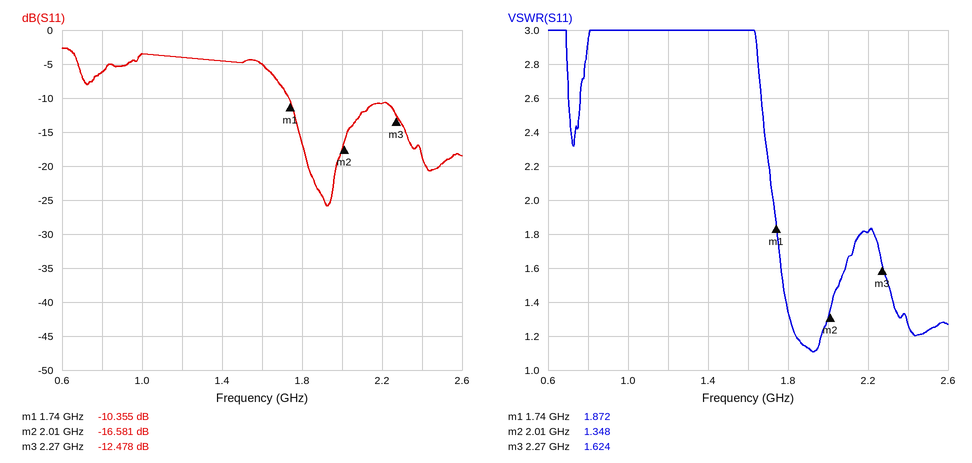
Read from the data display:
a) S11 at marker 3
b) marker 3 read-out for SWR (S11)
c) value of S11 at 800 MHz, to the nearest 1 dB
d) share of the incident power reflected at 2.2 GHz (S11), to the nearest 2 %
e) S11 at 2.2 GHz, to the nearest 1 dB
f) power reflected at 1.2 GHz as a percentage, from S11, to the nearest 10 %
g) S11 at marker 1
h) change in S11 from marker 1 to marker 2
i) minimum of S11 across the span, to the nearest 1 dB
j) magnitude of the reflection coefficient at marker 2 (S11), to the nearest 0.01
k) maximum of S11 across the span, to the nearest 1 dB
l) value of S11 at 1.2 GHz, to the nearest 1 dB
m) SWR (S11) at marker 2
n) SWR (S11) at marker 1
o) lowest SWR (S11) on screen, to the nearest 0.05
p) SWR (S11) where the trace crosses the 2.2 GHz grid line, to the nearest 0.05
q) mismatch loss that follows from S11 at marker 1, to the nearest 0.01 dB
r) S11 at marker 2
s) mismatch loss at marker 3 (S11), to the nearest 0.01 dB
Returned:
-12.478 dB
1.624
-6 dB
8 %
-11 dB
40 %
-10.355 dB
-6.226 dB
-26 dB
0.15
-3 dB
-4 dB
1.348
1.872
1.10
1.80
0.42 dB
-16.581 dB
0.25 dB
